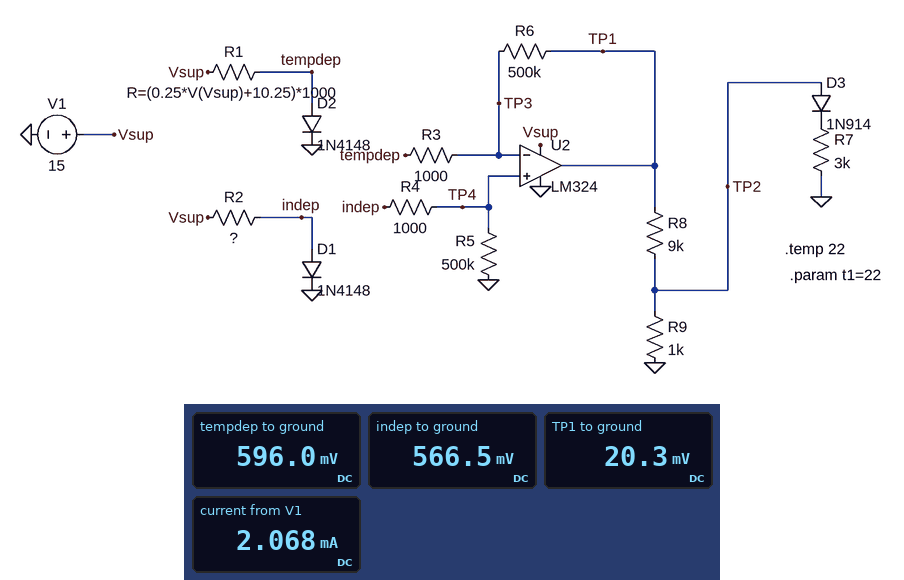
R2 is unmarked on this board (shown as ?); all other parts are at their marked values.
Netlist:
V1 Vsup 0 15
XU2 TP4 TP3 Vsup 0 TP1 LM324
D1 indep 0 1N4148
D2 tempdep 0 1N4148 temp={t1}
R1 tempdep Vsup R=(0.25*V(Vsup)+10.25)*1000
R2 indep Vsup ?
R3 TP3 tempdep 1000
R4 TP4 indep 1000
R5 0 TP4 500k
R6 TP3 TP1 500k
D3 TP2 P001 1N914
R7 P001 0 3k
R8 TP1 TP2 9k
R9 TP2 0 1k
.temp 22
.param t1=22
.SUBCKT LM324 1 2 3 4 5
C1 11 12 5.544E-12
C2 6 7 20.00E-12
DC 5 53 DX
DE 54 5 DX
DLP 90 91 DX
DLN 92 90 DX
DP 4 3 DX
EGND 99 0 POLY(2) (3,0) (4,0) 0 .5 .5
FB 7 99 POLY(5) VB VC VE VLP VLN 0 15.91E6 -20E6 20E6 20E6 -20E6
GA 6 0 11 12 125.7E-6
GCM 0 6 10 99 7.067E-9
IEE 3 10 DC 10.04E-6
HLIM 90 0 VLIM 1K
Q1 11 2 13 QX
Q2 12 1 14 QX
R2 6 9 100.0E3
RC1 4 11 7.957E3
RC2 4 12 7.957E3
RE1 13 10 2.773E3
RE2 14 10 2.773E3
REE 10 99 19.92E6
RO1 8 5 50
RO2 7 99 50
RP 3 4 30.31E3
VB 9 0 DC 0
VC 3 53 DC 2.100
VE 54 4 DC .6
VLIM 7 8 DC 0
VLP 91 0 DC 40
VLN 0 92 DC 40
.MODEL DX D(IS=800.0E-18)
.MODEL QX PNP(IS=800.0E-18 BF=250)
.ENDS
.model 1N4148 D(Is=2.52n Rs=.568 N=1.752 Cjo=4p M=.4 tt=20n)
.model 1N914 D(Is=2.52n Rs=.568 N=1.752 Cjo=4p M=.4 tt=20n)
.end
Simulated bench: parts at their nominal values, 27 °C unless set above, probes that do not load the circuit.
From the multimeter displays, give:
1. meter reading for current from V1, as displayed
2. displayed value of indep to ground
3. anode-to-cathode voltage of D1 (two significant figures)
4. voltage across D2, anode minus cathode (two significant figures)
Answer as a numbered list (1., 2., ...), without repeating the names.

1. 2.068 mA
2. 566.5 mV
3. 570 mV
4. 600 mV
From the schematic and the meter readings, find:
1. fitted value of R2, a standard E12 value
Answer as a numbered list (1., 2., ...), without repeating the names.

1. 27 kΩ
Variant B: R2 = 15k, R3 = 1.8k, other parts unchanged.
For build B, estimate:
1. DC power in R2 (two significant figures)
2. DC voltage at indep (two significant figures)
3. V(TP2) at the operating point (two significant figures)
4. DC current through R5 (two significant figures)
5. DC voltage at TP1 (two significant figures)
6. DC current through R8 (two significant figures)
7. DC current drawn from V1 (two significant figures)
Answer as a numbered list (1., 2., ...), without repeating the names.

1. 14 mW
2. 590 mV
3. 8.7 mV
4. 1.2 µA
5. 87 mV
6. 8.7 µA
7. 2.5 mA
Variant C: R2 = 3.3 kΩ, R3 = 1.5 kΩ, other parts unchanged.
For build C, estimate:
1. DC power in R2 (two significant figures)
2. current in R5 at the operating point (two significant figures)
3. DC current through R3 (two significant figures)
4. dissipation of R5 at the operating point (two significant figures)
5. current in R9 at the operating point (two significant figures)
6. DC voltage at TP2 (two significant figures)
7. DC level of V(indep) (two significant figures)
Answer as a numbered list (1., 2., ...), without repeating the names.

1. 62 mW
2. 1.3 µA
3. 26 µA
4. 870 nW
5. 1.2 mA
6. 1.2 V
7. 660 mV
